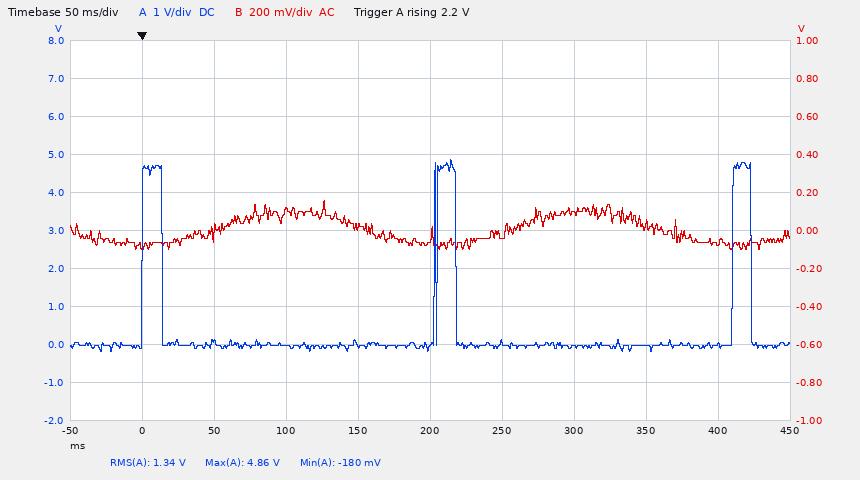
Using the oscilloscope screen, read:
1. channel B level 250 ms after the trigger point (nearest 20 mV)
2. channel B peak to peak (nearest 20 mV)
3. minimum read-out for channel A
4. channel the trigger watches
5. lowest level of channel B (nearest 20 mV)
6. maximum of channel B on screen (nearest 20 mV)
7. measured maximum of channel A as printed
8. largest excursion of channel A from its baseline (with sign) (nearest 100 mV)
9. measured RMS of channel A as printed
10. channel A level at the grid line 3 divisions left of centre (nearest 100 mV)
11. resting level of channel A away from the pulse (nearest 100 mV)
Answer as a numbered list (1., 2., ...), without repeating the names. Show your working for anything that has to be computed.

1. -20 mV
2. 160 mV − (-100 mV) = 260 mV
3. -180 mV
4. channel A
5. -100 mV
6. 160 mV
7. 4.86 V
8. +4.9 V
9. 1.34 V
10. 100 mV
11. 0.0 V
